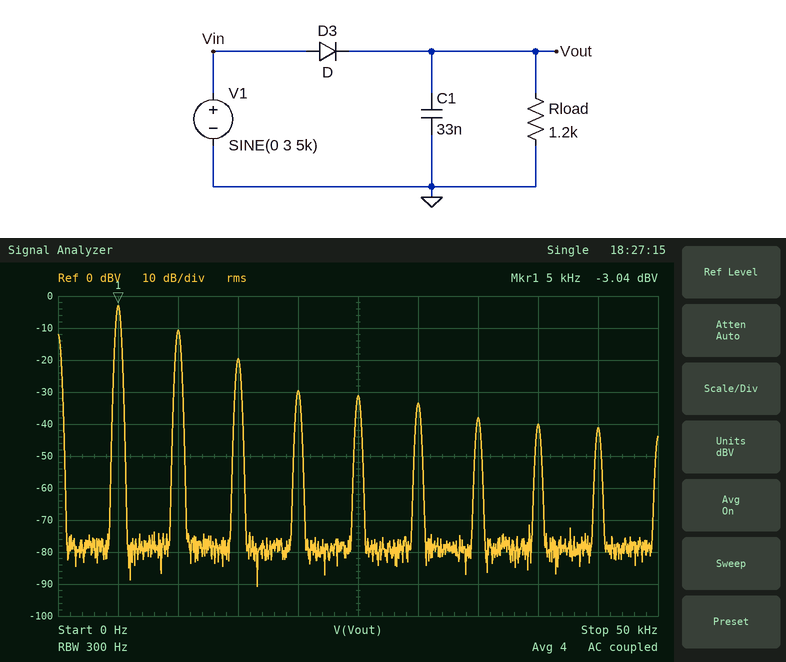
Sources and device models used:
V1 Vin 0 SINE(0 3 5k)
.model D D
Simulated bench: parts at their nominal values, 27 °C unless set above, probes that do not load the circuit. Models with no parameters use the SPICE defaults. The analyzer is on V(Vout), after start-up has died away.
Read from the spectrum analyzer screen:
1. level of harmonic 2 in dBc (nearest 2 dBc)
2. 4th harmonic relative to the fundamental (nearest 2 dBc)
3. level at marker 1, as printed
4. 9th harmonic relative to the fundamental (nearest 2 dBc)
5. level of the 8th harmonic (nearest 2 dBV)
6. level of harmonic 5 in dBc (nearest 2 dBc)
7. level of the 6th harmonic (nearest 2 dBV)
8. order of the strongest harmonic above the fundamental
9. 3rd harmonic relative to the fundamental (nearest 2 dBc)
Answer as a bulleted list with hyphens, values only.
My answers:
- -8 dBc
- -26 dBc
- -3.04 dBV
- -38 dBc
- -40 dBV
- -28 dBc
- -34 dBV
- 2
- -16 dBc
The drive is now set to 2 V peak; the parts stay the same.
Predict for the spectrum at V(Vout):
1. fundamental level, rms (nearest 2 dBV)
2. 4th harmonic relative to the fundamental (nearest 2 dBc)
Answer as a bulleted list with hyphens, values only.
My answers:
- -8 dBV
- -24 dBc
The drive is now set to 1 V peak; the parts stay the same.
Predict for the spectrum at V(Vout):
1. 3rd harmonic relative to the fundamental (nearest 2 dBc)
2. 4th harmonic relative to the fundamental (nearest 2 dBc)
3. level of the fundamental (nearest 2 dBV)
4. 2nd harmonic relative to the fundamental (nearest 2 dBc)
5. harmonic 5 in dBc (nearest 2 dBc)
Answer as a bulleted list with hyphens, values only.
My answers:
- -12 dBc
- -18 dBc
- -20 dBV
- -6 dBc
- -24 dBc
